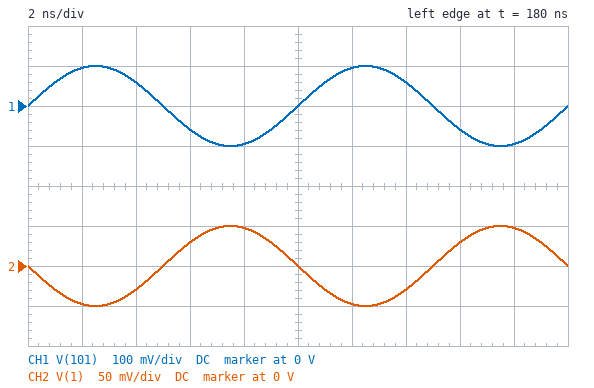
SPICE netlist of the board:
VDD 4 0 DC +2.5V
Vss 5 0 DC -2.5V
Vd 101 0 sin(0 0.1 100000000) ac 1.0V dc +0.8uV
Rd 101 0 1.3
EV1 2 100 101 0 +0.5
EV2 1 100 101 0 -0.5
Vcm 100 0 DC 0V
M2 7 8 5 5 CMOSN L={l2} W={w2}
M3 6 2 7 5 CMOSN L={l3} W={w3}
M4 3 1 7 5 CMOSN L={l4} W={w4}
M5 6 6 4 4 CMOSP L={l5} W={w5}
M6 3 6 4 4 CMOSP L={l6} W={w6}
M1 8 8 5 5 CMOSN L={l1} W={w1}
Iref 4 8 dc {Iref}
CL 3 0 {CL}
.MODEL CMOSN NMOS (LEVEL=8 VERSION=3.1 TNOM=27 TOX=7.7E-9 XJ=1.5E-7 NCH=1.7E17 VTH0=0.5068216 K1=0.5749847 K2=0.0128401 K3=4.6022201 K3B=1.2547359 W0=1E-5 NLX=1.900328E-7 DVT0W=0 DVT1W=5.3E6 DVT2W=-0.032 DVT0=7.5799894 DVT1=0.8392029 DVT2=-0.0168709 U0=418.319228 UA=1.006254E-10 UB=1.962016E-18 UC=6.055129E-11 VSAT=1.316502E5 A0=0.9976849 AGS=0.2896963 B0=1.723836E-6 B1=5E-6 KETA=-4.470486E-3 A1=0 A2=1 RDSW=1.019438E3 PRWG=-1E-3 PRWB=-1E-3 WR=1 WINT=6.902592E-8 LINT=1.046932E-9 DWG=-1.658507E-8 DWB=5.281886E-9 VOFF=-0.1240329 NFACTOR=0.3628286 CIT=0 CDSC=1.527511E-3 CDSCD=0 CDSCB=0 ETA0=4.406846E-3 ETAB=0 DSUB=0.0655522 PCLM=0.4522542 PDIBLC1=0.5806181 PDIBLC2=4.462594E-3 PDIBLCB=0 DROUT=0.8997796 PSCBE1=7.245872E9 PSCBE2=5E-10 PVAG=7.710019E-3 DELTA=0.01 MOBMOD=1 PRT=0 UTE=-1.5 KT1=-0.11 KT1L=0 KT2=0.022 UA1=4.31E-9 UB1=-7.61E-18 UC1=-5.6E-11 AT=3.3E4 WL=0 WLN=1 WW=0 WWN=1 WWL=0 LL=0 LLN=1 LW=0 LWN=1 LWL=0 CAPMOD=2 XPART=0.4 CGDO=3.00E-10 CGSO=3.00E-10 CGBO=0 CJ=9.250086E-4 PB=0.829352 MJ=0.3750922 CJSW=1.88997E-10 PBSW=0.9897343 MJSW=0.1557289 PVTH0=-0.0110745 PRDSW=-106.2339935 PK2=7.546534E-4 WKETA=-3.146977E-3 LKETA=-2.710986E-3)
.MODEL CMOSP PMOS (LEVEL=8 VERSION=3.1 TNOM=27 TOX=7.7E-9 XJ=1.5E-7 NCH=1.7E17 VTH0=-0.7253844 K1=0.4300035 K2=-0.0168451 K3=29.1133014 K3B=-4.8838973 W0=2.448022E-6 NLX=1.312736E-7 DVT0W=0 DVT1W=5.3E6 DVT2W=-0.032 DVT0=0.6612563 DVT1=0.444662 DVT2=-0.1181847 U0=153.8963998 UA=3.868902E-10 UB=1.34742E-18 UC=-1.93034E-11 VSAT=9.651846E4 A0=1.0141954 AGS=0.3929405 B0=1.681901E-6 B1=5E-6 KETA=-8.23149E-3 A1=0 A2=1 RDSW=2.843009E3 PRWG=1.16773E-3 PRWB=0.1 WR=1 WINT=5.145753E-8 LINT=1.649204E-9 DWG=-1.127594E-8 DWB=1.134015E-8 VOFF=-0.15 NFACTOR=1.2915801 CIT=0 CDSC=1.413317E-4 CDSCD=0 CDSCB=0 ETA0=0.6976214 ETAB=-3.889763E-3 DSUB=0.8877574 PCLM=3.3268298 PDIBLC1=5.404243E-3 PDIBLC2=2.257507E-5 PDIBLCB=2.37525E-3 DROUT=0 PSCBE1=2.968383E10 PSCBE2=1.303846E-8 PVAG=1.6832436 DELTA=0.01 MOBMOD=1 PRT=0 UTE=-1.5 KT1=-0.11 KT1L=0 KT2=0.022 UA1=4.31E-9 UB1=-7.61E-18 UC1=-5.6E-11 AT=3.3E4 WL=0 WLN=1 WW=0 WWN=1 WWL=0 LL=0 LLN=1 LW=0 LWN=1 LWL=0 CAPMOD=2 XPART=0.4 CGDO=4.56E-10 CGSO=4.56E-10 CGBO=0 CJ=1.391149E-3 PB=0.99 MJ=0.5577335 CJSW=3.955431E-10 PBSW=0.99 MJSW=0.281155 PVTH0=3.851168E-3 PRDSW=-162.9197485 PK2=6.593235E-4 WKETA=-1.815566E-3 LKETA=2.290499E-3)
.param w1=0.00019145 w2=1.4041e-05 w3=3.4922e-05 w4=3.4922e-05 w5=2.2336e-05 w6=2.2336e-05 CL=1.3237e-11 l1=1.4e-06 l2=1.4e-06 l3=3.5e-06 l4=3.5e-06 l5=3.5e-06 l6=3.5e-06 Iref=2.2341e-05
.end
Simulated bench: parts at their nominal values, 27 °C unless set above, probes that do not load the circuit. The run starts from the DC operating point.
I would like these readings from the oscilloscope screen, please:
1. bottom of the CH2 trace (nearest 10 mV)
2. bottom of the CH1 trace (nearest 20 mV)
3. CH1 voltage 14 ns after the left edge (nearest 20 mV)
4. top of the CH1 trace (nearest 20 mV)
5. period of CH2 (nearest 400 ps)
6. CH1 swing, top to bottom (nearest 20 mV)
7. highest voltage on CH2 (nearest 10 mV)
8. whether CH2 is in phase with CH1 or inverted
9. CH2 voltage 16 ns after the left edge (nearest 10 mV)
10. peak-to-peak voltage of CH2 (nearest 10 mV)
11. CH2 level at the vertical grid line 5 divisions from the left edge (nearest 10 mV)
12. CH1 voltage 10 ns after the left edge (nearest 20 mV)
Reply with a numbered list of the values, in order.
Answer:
1. -50 mV
2. -100 mV
3. 60 mV
4. 100 mV
5. 10.0 ns
6. 200 mV
7. 50 mV
8. inverted
9. 30 mV
10. 100 mV
11. 0 V
12. 0 V
